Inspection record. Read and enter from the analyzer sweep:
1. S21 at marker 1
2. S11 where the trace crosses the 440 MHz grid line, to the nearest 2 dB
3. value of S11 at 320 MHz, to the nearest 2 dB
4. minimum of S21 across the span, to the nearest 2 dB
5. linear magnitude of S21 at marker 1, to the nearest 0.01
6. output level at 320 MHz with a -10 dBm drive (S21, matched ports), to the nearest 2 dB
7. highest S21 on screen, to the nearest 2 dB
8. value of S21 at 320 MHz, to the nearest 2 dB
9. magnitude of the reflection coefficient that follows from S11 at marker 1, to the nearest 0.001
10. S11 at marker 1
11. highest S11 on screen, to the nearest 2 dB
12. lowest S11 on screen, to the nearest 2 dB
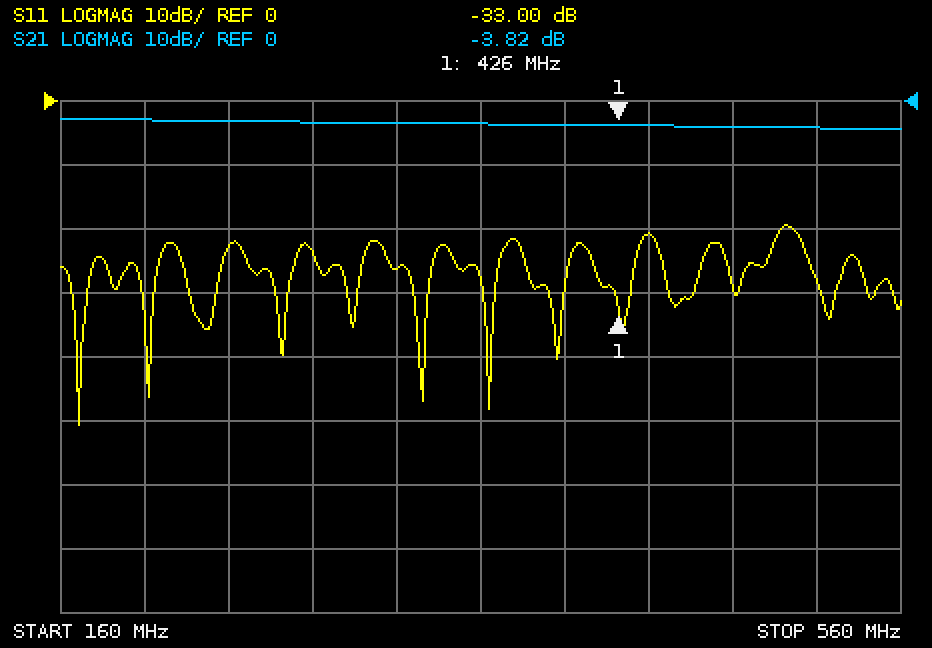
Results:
-3.82 dB
-20 dB
-26 dB
-4 dB
0.64
-14 dBm
-2 dB
-4 dB
0.022
-33.00 dB
-20 dB
-50 dB
